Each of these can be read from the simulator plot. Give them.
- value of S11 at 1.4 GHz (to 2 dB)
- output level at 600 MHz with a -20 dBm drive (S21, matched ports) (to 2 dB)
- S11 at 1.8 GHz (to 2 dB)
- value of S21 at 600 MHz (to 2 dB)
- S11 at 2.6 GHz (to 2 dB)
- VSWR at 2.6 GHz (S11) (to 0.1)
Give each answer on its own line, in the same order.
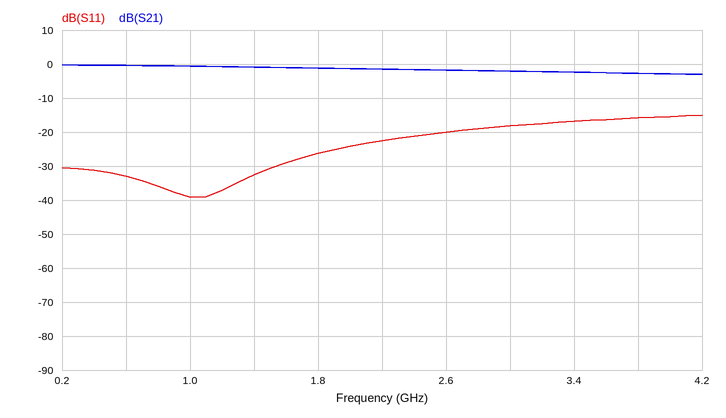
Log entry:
-32 dB
-20 dBm
-26 dB
0 dB
-20 dB
1.2
